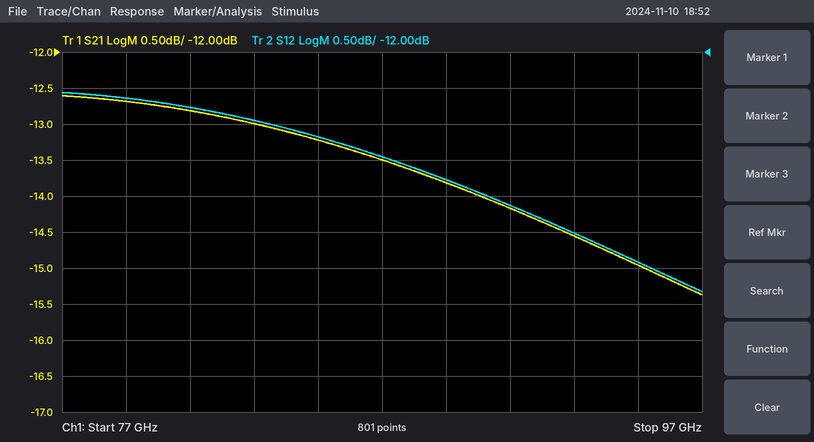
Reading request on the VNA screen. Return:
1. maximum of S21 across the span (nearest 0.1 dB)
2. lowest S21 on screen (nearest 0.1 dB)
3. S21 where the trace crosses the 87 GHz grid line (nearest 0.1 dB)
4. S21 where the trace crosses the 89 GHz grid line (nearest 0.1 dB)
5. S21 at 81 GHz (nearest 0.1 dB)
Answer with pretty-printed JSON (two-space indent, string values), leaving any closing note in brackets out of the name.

{
  "maximum of S21 across the span": "-12.6 dB",
  "lowest S21 on screen": "-15.4 dB",
  "S21 where the trace crosses the 87 GHz grid line": "-13.5 dB",
  "S21 where the trace crosses the 89 GHz grid line": "-13.8 dB",
  "S21 at 81 GHz": "-12.8 dB"
}
